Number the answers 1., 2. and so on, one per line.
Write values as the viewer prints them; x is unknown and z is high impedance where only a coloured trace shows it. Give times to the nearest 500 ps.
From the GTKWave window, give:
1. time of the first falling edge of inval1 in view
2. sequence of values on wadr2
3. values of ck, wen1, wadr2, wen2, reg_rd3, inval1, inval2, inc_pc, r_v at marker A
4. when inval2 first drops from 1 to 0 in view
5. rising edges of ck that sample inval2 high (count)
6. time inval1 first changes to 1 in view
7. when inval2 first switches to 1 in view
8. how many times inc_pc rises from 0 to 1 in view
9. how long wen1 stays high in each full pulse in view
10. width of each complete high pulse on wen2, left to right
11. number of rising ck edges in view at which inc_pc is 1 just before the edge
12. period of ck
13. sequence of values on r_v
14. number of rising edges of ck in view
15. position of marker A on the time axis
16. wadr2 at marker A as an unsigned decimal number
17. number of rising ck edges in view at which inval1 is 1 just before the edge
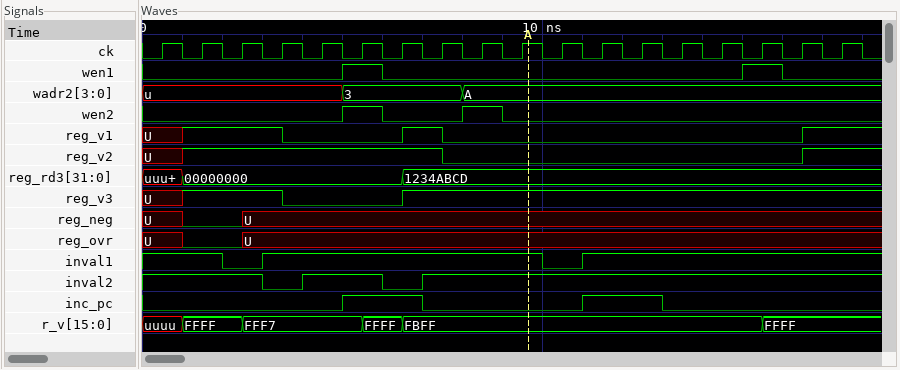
1. 2000 ps
2. u, 3, A
3. ck=1, wen1=0, wadr2=A, wen2=0, reg_rd3=1234ABCD, inval1=1, inval2=1, inc_pc=0, r_v=FBFF
4. 3000 ps
5. 16
6. 3000 ps
7. 4000 ps
8. 2
9. 1000 ps, 1000 ps
10. 1000 ps, 1000 ps
11. 4
12. 1000 ps
13. uuuu, FFFF, FFF7, FFFF, FBFF, FFFF
14. 18
15. 9500 ps
16. 10
17. 16
